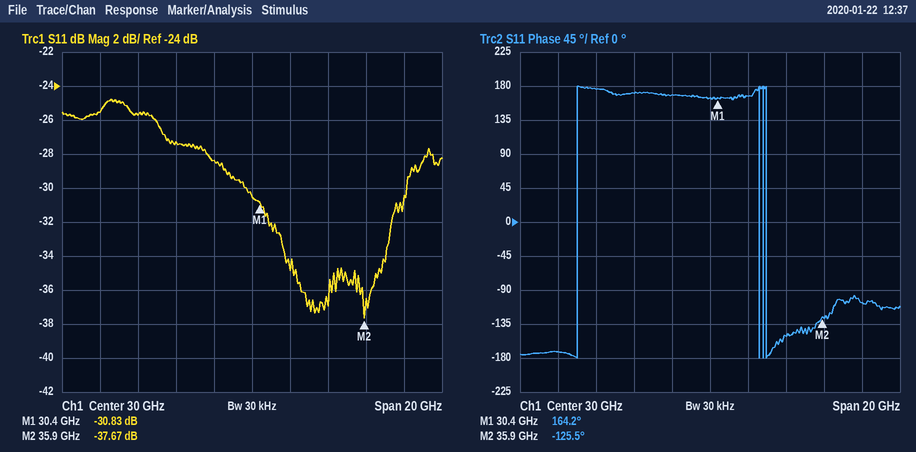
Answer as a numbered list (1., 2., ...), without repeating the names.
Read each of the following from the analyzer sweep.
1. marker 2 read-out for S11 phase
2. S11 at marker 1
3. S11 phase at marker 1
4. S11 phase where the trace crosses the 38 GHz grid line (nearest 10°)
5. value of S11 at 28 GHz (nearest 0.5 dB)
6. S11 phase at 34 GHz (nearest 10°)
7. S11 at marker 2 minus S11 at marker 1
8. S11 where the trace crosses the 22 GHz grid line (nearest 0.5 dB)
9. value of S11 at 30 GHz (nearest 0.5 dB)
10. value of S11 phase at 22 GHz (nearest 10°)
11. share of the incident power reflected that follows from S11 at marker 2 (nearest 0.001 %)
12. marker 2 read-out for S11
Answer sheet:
1. -125.5°
2. -30.83 dB
3. 164.2°
4. -110°
5. -28.5 dB
6. -150°
7. -6.84 dB
8. -25.5 dB
9. -30.5 dB
10. -170°
11. 0.017 %
12. -37.67 dB
